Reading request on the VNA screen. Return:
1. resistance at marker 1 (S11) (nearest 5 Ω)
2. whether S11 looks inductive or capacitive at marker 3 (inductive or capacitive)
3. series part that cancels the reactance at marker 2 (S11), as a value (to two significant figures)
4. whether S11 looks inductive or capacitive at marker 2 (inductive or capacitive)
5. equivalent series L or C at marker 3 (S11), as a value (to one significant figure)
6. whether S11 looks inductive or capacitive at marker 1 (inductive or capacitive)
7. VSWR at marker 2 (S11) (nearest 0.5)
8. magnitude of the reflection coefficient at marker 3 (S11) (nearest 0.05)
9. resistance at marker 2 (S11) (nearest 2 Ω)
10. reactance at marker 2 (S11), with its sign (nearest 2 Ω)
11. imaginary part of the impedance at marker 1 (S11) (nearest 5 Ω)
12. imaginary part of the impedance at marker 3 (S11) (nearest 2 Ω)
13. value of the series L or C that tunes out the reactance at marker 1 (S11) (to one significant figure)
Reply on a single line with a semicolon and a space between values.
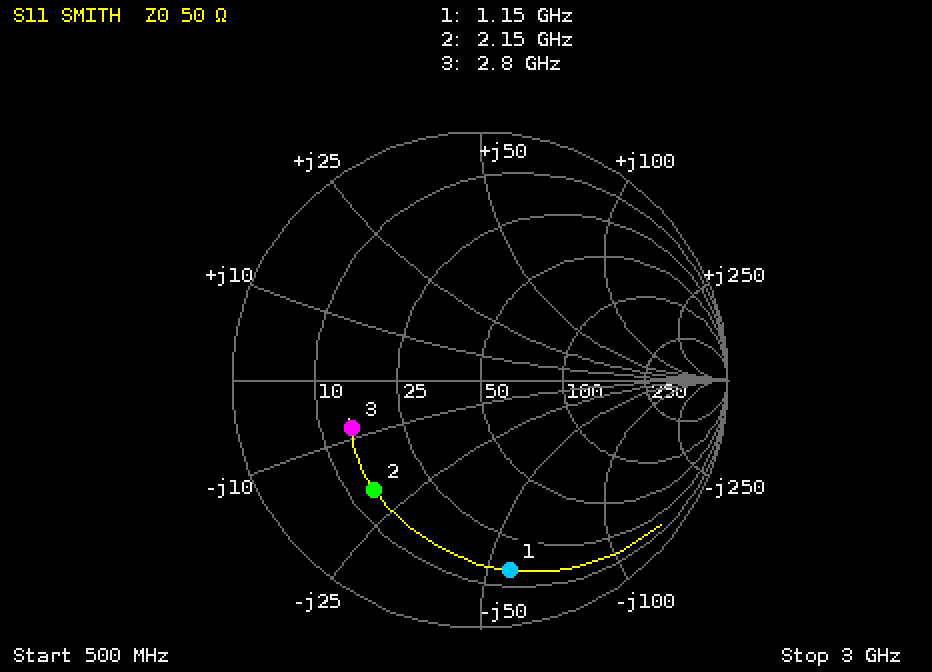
15 Ω; capacitive; 1.5 nH; capacitive; 7 pF; capacitive; 4.0; 0.55; 14 Ω; -20 Ω; -55 Ω; -8 Ω; 8 nH
